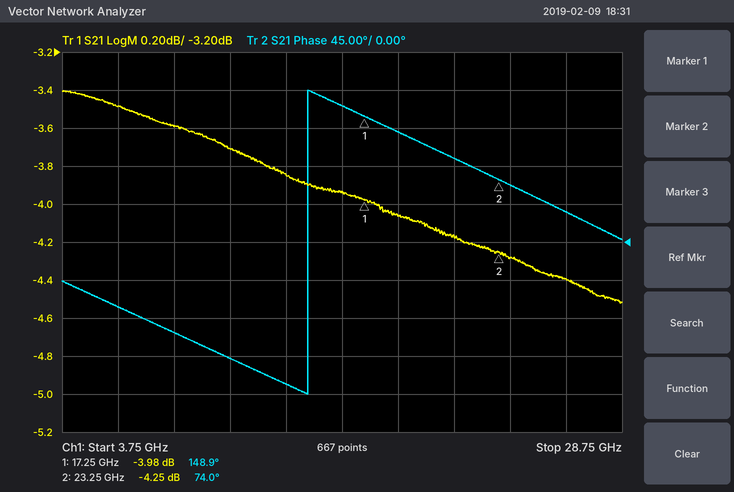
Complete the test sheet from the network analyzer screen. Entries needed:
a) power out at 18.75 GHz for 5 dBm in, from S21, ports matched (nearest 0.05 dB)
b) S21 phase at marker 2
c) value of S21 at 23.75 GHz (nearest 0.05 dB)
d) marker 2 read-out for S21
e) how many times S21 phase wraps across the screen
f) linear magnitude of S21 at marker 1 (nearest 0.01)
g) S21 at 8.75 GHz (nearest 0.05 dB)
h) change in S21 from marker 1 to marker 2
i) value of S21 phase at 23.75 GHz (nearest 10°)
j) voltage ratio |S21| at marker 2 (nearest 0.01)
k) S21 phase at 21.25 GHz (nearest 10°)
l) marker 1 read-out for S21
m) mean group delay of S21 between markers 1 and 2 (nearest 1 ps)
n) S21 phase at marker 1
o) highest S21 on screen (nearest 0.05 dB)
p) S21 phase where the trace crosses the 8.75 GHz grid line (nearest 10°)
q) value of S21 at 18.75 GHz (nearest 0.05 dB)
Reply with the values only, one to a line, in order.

0.95 dBm
74.0°
-4.30 dB
-4.25 dB
1
0.63
-3.60 dB
-0.27 dB
70°
0.61
100°
-3.98 dB
35 ps
148.9°
-3.40 dB
-110°
-4.05 dB
